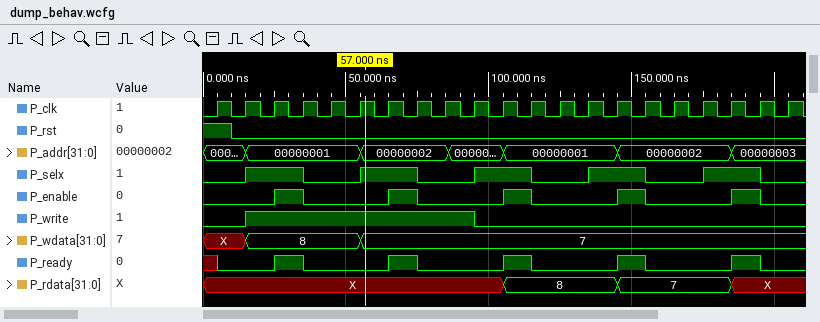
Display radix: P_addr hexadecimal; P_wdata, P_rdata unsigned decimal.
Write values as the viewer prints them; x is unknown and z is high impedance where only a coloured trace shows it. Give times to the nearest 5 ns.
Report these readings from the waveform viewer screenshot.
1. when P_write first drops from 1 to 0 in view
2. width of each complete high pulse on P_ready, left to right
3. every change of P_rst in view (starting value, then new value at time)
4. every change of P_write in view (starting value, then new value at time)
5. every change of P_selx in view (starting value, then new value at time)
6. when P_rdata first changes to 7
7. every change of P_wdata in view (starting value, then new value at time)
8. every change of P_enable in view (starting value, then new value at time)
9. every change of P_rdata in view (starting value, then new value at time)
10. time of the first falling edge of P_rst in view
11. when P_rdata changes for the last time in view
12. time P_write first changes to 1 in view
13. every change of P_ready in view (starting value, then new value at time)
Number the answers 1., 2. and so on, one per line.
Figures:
1. 95 ns
2. 10 ns, 10 ns, 10 ns, 10 ns, 10 ns
3. 1, 0 at 10 ns
4. 0, 1 at 15 ns, 0 at 95 ns
5. 0, 1 at 15 ns, 0 at 35 ns, 1 at 55 ns, 0 at 75 ns, 1 at 95 ns, 0 at 115 ns, 1 at 135 ns, 0 at 155 ns, 1 at 175 ns, 0 at 195 ns
6. 145 ns
7. X, 8 at 15 ns, 7 at 55 ns
8. 0, 1 at 25 ns, 0 at 35 ns, 1 at 65 ns, 0 at 75 ns, 1 at 105 ns, 0 at 115 ns, 1 at 145 ns, 0 at 155 ns, 1 at 185 ns, 0 at 195 ns
9. X, 8 at 105 ns, 7 at 145 ns, X at 185 ns
10. 10 ns
11. 185 ns
12. 15 ns
13. x, 0 at 5 ns, 1 at 25 ns, 0 at 35 ns, 1 at 65 ns, 0 at 75 ns, 1 at 105 ns, 0 at 115 ns, 1 at 145 ns, 0 at 155 ns, 1 at 185 ns, 0 at 195 ns
